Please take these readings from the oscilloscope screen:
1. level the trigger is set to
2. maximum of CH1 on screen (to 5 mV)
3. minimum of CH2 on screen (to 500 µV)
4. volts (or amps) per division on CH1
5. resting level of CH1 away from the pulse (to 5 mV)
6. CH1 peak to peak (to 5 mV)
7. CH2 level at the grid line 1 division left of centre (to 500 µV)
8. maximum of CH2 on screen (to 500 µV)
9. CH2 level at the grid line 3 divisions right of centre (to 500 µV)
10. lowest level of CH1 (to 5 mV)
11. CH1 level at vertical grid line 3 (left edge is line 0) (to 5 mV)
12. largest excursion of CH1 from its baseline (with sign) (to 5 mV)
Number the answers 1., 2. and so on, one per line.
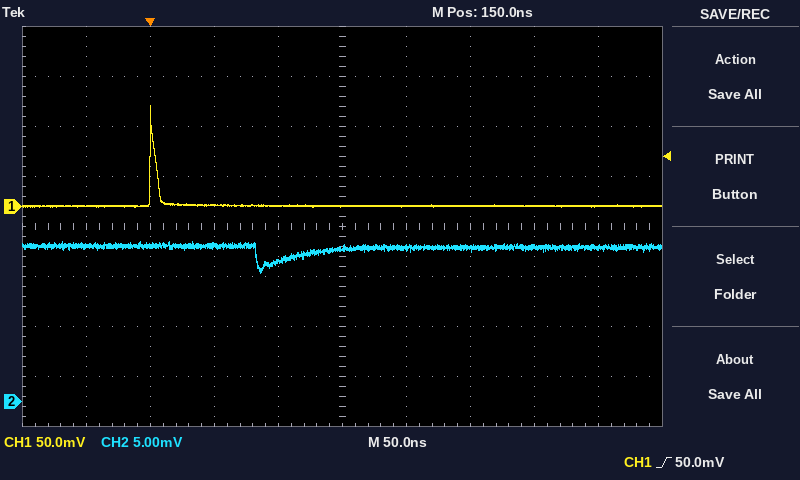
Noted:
1. 50.0 mV
2. 100 mV
3. 13.0 mV
4. 50 mV
5. 0 mV
6. 100 mV
7. 14.0 mV
8. 16.0 mV
9. 15.5 mV
10. 0 mV
11. 0 mV
12. +100 mV
